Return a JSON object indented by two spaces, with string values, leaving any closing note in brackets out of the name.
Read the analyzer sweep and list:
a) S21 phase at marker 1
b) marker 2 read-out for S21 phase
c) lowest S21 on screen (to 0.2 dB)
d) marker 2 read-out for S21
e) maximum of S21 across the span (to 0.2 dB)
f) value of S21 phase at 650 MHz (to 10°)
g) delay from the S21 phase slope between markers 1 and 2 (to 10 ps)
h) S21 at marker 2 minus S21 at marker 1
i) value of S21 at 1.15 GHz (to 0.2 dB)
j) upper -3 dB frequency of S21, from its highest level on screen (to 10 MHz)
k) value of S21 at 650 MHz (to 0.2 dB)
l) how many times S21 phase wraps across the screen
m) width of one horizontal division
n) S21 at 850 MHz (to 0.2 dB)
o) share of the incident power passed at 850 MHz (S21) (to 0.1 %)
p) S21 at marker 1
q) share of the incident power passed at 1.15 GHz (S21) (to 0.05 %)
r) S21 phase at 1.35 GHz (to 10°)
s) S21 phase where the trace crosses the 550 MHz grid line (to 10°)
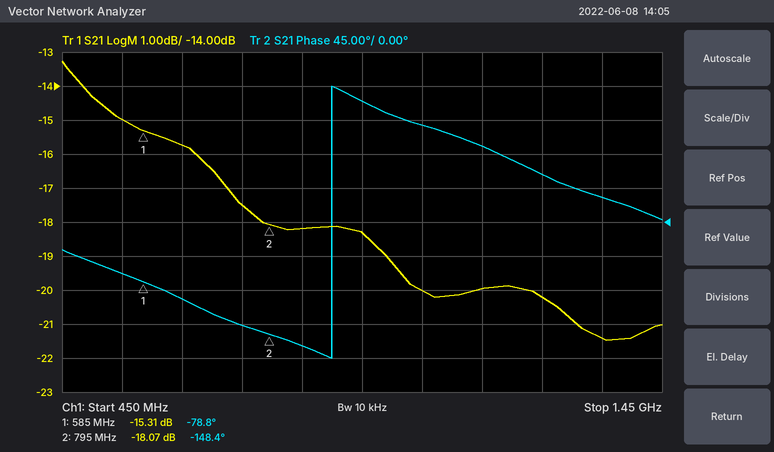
{
  "S21 phase at marker 1": "-78.8°",
  "marker 2 read-out for S21 phase": "-148.4°",
  "lowest S21 on screen": "-21.4 dB",
  "marker 2 read-out for S21": "-18.07 dB",
  "maximum of S21 across the span": "-13.2 dB",
  "value of S21 phase at 650 MHz": "-100°",
  "delay from the S21 phase slope between markers 1 and 2": "920 ps",
  "S21 at marker 2 minus S21 at marker 1": "-2.76 dB",
  "value of S21 at 1.15 GHz": "-20.0 dB",
  "upper -3 dB frequency of S21, from its highest level on screen": "690 MHz",
  "value of S21 at 650 MHz": "-15.8 dB",
  "how many times S21 phase wraps across the screen": "1",
  "width of one horizontal division": "100 MHz",
  "S21 at 850 MHz": "-18.2 dB",
  "share of the incident power passed at 850 MHz (S21)": "1.5 %",
  "S21 at marker 1": "-15.31 dB",
  "share of the incident power passed at 1.15 GHz (S21)": "1.00 %",
  "S21 phase at 1.35 GHz": "30°",
  "S21 phase where the trace crosses the 550 MHz grid line": "-70°"
}
